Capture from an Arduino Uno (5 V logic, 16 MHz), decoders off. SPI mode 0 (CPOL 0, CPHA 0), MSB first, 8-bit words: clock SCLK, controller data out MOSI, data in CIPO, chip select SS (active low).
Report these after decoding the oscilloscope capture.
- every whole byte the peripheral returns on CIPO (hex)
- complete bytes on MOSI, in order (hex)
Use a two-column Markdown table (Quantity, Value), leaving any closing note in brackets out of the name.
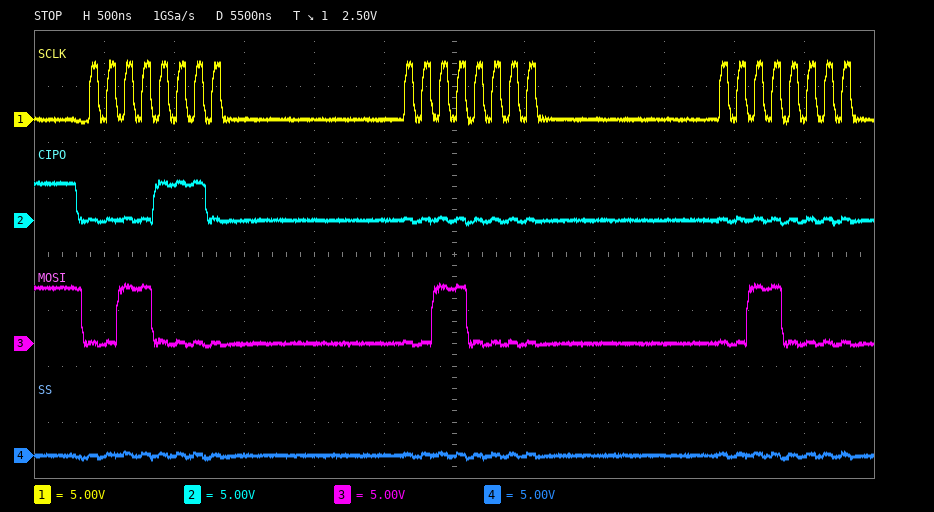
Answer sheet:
| Quantity | Value |
|---|---|
| every whole byte the peripheral returns on CIPO | 0x0E 0x00 0x00 |
| complete bytes on MOSI, in order | 0x30 0x30 0x30 |
